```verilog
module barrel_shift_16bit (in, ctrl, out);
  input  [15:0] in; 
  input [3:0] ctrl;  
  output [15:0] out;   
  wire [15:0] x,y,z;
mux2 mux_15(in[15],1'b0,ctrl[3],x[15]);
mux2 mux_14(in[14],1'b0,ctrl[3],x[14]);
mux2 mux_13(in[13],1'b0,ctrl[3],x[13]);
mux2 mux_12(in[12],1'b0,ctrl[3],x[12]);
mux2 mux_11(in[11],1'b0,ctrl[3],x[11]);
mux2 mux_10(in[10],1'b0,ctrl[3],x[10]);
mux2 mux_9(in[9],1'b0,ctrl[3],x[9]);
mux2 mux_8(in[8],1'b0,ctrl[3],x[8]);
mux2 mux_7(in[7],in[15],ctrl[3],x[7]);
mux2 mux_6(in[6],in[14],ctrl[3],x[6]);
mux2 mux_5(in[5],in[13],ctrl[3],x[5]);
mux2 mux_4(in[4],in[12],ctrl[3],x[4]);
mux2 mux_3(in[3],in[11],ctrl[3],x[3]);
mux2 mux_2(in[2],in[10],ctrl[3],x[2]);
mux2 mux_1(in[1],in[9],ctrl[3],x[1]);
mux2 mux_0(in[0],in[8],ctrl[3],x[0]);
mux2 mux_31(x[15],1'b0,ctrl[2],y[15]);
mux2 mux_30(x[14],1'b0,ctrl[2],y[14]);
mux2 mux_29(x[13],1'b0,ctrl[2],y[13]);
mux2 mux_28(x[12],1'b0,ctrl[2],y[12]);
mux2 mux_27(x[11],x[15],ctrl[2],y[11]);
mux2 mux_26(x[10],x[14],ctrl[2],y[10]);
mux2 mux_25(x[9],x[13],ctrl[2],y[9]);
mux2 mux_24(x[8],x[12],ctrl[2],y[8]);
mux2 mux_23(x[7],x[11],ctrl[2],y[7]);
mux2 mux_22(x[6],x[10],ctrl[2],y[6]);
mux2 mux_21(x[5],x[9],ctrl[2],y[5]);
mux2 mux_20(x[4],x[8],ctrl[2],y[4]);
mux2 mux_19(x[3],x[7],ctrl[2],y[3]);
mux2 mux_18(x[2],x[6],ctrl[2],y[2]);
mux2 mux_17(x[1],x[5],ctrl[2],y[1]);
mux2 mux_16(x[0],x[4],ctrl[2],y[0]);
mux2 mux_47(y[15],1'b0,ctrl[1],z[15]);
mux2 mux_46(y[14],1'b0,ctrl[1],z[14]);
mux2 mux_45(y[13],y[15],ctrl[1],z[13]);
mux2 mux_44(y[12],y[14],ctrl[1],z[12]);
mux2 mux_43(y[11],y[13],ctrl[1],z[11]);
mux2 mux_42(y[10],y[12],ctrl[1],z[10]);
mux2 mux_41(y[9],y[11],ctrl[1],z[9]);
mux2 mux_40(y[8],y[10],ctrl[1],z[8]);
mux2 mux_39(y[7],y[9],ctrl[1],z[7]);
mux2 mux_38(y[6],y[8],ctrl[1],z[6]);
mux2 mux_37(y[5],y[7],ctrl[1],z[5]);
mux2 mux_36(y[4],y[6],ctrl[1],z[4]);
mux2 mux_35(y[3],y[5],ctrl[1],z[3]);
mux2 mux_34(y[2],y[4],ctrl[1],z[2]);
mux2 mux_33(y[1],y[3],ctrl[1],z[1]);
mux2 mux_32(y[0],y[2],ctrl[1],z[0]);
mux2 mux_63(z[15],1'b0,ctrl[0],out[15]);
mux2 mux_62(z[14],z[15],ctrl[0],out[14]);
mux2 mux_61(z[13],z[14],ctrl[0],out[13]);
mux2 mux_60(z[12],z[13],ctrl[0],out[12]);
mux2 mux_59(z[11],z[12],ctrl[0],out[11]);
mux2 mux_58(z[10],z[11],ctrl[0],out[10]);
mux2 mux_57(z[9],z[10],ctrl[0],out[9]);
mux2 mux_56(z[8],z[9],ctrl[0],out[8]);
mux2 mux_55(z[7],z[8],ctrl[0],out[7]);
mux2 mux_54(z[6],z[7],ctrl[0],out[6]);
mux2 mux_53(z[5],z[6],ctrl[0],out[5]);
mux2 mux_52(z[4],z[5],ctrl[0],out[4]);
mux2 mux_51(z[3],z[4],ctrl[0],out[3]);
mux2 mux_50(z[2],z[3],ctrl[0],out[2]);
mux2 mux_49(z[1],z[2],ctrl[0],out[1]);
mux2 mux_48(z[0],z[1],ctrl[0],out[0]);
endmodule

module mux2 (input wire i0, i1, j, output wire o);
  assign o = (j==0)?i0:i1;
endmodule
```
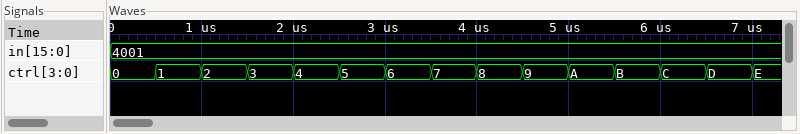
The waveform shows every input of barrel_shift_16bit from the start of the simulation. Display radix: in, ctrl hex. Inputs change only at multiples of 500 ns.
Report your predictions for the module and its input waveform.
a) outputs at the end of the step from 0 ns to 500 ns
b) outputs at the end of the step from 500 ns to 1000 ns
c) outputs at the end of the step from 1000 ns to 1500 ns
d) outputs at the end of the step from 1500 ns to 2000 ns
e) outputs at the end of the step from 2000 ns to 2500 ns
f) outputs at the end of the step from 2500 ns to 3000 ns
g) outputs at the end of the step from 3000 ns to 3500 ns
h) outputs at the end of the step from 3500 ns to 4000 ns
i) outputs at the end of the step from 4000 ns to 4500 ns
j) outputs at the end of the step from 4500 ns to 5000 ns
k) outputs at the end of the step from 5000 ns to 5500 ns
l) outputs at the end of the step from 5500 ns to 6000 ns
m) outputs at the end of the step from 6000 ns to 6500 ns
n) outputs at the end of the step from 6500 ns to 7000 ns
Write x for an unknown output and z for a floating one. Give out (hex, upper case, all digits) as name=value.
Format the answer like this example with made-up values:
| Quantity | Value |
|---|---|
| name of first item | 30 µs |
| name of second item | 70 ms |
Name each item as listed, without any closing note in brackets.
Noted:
| Quantity | Value |
|---|---|
| outputs at the end of the step from 0 ns to 500 ns | out=4001 |
| outputs at the end of the step from 500 ns to 1000 ns | out=2000 |
| outputs at the end of the step from 1000 ns to 1500 ns | out=1000 |
| outputs at the end of the step from 1500 ns to 2000 ns | out=0800 |
| outputs at the end of the step from 2000 ns to 2500 ns | out=0400 |
| outputs at the end of the step from 2500 ns to 3000 ns | out=0200 |
| outputs at the end of the step from 3000 ns to 3500 ns | out=0100 |
| outputs at the end of the step from 3500 ns to 4000 ns | out=0080 |
| outputs at the end of the step from 4000 ns to 4500 ns | out=0040 |
| outputs at the end of the step from 4500 ns to 5000 ns | out=0020 |
| outputs at the end of the step from 5000 ns to 5500 ns | out=0010 |
| outputs at the end of the step from 5500 ns to 6000 ns | out=0008 |
| outputs at the end of the step from 6000 ns to 6500 ns | out=0004 |
| outputs at the end of the step from 6500 ns to 7000 ns | out=0002 |
